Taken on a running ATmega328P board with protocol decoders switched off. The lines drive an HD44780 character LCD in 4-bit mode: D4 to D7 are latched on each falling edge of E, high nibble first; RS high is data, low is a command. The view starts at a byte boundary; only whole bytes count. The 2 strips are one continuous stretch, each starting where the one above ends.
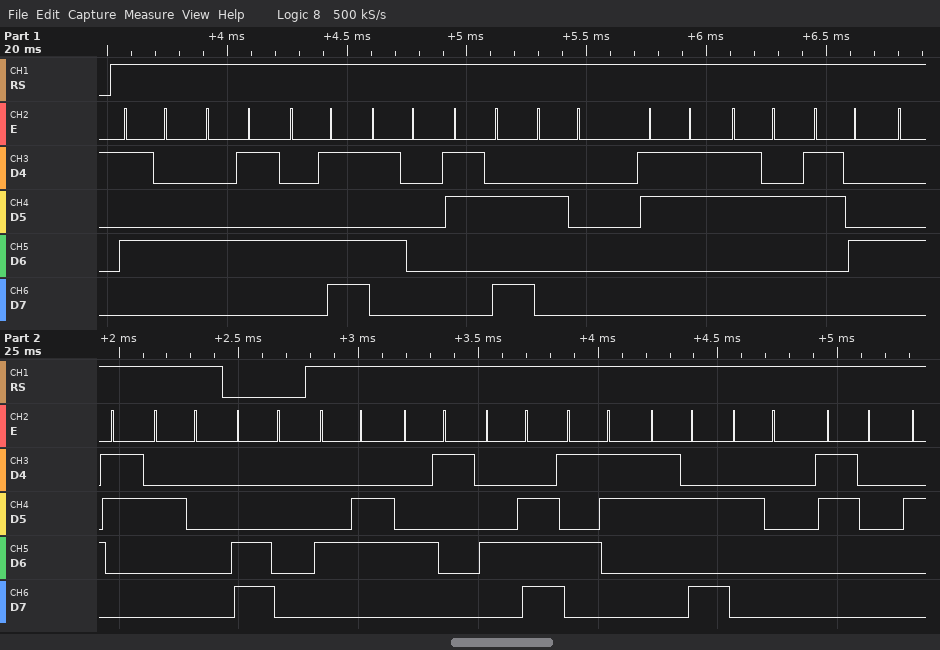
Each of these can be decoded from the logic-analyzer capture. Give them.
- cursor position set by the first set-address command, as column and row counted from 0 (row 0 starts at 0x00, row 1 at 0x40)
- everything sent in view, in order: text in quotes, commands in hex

column 0, row 1
"TEMP: 324C " 0xC0 "FANS: 0"
